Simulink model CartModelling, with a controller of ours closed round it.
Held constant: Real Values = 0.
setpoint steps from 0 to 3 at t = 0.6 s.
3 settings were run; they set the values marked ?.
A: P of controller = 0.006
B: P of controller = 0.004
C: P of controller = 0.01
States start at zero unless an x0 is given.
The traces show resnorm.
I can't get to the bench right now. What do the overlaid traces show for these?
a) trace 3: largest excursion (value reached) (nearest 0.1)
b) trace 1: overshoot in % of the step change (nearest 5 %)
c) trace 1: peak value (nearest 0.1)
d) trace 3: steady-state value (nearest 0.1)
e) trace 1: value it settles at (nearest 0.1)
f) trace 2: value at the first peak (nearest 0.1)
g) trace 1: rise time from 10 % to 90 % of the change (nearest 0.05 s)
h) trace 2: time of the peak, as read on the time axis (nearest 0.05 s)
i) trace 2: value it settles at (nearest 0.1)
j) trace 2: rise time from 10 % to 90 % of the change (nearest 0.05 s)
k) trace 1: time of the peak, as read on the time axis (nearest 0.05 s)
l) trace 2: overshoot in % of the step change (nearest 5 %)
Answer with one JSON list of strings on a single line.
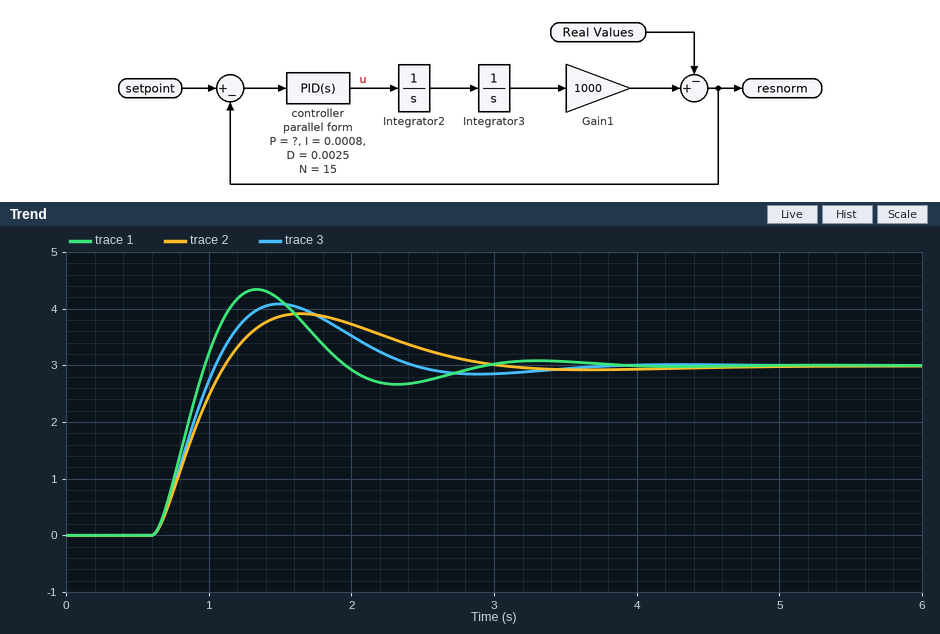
["4.1", "45 %", "4.3", "3.0", "3.0", "3.9", "0.25 s", "1.65 s", "3.0", "0.35 s", "1.35 s", "30 %"]
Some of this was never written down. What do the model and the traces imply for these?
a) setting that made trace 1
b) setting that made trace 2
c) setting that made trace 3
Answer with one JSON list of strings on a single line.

["C", "B", "A"]
